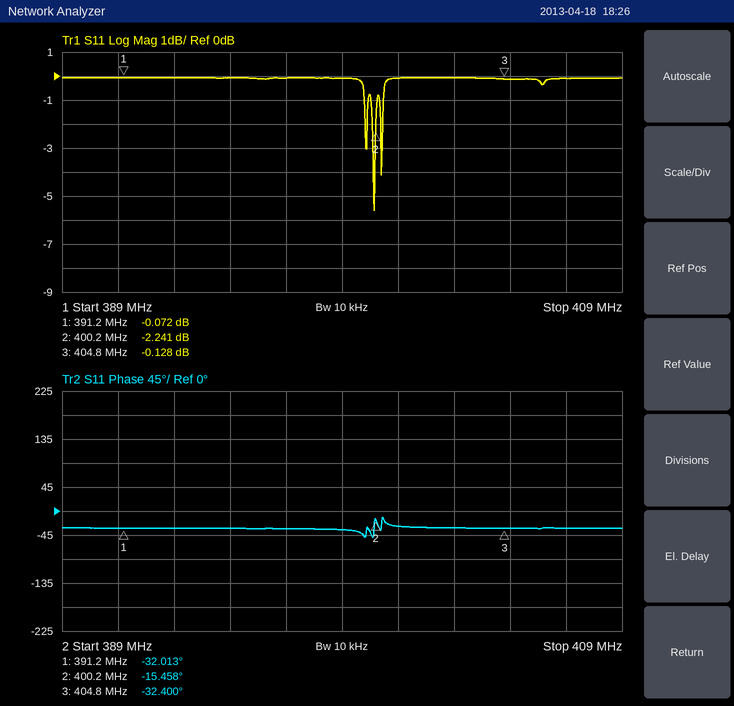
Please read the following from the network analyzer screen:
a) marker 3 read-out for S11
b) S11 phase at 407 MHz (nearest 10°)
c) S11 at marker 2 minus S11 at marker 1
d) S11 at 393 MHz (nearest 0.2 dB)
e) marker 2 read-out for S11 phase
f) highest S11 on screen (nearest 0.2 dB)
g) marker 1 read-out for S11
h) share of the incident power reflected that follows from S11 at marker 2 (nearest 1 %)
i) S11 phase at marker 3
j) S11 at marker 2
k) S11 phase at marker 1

-0.128 dB
-30°
-2.169 dB
0.0 dB
-15.458°
0.0 dB
-0.072 dB
60 %
-32.400°
-2.241 dB
-32.013°
